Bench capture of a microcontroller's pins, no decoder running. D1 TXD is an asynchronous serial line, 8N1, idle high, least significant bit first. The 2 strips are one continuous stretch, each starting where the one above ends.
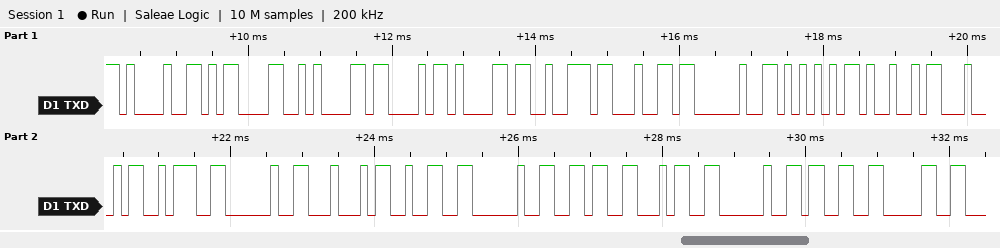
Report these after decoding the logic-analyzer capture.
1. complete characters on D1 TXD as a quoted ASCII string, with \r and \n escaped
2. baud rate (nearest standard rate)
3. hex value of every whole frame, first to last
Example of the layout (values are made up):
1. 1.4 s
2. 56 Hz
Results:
1. "!\r\nCard UID: D2 64 30"
2. 9600 baud
3. 21 0D 0A 43 61 72 64 20 55 49 44 3A 20 44 32 20 36 34 20 33 30
